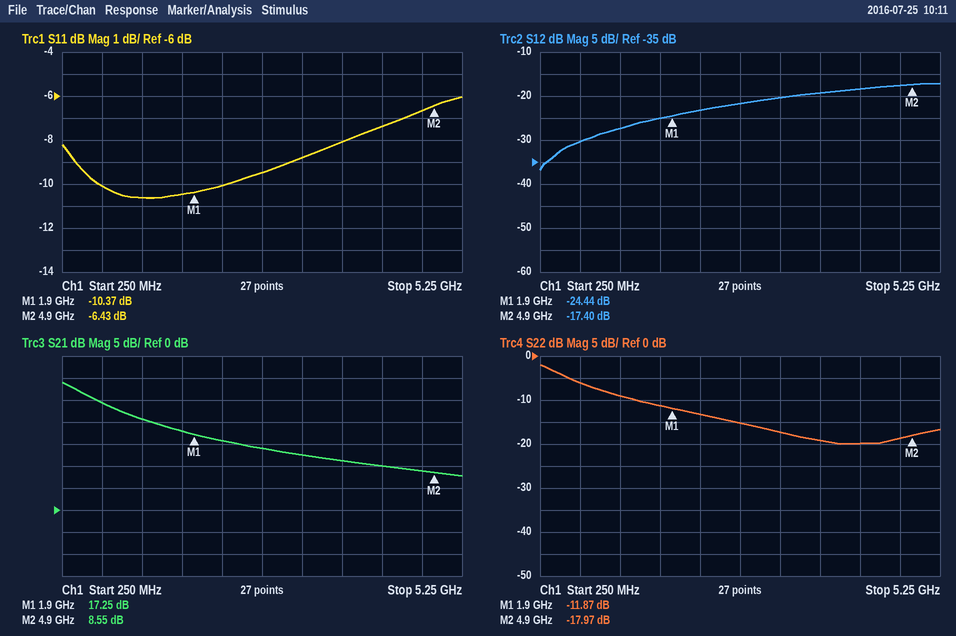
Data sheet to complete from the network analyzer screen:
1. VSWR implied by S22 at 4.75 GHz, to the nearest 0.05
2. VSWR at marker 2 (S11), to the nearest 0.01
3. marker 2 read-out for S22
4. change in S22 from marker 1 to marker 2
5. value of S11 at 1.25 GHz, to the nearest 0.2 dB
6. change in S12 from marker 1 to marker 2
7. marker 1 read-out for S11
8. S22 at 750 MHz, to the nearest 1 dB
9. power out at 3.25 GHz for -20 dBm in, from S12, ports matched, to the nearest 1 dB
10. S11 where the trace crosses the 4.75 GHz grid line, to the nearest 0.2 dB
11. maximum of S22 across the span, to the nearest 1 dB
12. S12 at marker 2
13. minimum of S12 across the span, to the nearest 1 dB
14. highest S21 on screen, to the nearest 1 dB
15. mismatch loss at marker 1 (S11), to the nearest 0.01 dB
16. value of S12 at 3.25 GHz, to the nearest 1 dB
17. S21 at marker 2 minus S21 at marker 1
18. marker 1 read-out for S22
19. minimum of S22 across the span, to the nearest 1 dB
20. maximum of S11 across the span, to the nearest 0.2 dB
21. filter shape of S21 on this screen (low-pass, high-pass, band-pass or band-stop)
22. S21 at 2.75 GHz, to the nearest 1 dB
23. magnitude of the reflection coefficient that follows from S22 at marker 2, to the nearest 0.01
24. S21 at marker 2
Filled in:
1.25
2.82
-17.97 dB
-6.10 dB
-10.6 dB
7.04 dB
-10.37 dB
-6 dB
-40 dBm
-6.6 dB
-2 dB
-17.40 dB
-37 dB
29 dB
0.42 dB
-20 dB
-8.70 dB
-11.87 dB
-20 dB
-6.0 dB
low-pass
14 dB
0.13
8.55 dB
